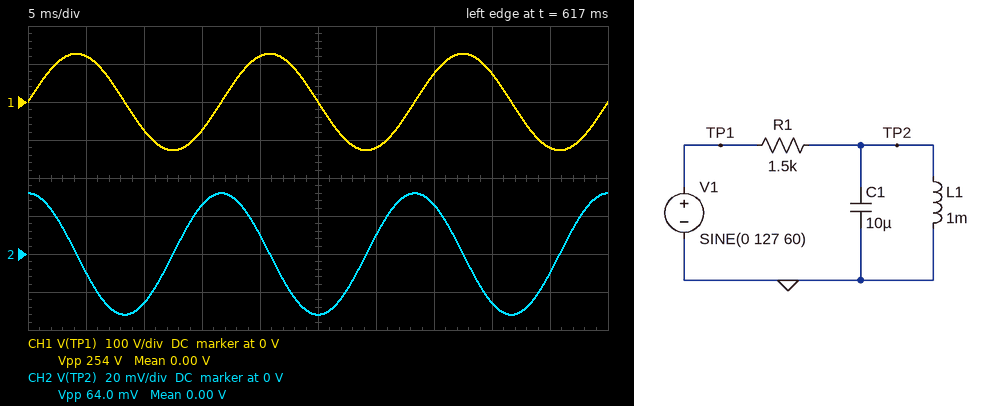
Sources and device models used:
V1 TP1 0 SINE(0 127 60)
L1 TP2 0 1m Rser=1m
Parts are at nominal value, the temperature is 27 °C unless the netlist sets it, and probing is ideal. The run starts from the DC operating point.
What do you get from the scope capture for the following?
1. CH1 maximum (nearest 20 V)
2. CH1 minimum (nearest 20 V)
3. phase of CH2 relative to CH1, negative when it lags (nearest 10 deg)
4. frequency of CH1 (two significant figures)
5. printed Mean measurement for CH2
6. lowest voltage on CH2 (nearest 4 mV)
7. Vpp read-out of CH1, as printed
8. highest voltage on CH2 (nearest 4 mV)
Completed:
120 V
-120 V
90 deg
60 Hz
0.00 V
-32 mV
254 V
32 mV
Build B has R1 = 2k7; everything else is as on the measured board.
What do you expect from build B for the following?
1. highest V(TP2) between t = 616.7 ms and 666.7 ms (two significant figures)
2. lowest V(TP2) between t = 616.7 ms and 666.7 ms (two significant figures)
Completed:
18 mV
-18 mV
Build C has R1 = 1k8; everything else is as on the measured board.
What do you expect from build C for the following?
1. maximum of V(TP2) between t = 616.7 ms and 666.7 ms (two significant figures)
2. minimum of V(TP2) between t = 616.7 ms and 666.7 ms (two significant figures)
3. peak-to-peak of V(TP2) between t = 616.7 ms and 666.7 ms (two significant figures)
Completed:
27 mV
-27 mV
53 mV
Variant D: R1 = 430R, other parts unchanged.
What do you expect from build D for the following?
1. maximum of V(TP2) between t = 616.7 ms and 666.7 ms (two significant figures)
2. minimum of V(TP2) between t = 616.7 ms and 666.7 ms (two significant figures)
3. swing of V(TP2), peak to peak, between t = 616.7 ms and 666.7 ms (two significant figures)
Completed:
110 mV
-110 mV
220 mV
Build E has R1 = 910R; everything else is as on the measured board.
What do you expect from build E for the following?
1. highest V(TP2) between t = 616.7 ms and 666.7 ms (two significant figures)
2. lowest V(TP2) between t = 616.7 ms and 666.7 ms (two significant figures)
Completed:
53 mV
-53 mV
